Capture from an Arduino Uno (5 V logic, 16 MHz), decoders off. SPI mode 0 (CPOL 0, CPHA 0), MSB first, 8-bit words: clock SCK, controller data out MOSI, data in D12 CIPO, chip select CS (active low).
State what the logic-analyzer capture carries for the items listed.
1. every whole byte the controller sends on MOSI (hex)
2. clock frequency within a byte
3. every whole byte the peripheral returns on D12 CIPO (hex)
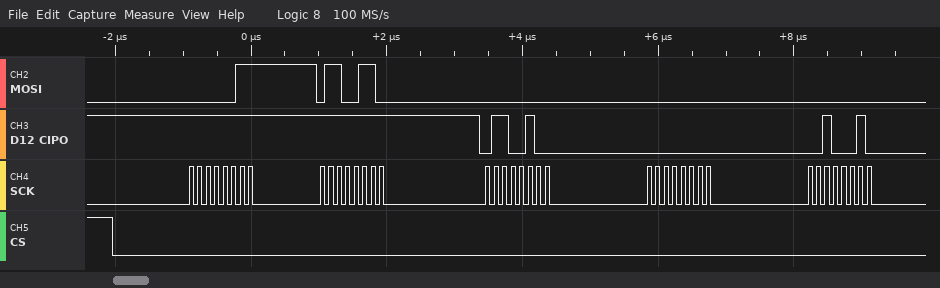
03 66 00 00 00
8 MHz
FF FF 64 00 22
